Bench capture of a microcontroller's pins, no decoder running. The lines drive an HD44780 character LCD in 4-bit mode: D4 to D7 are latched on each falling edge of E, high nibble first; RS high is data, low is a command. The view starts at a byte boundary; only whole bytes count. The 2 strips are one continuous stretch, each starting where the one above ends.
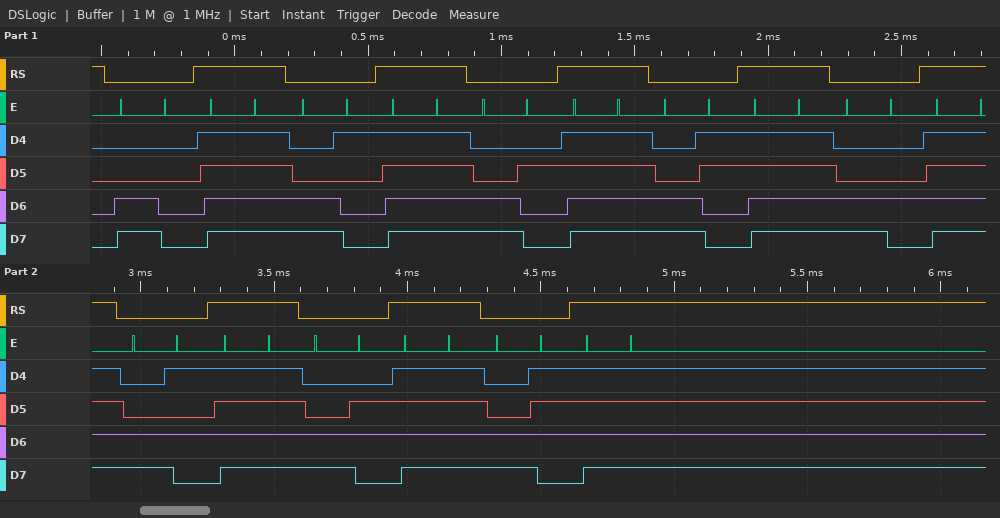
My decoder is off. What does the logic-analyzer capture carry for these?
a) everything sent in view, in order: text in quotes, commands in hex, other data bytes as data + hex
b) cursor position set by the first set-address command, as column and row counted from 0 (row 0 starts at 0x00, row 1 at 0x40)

0xC0 data FF 0xC1 data FF 0xC2 data FF 0xC3 data FF 0xC4 data FF 0xC5 data FF 0xC6 data FF 0xC7 data FF
column 0, row 1
